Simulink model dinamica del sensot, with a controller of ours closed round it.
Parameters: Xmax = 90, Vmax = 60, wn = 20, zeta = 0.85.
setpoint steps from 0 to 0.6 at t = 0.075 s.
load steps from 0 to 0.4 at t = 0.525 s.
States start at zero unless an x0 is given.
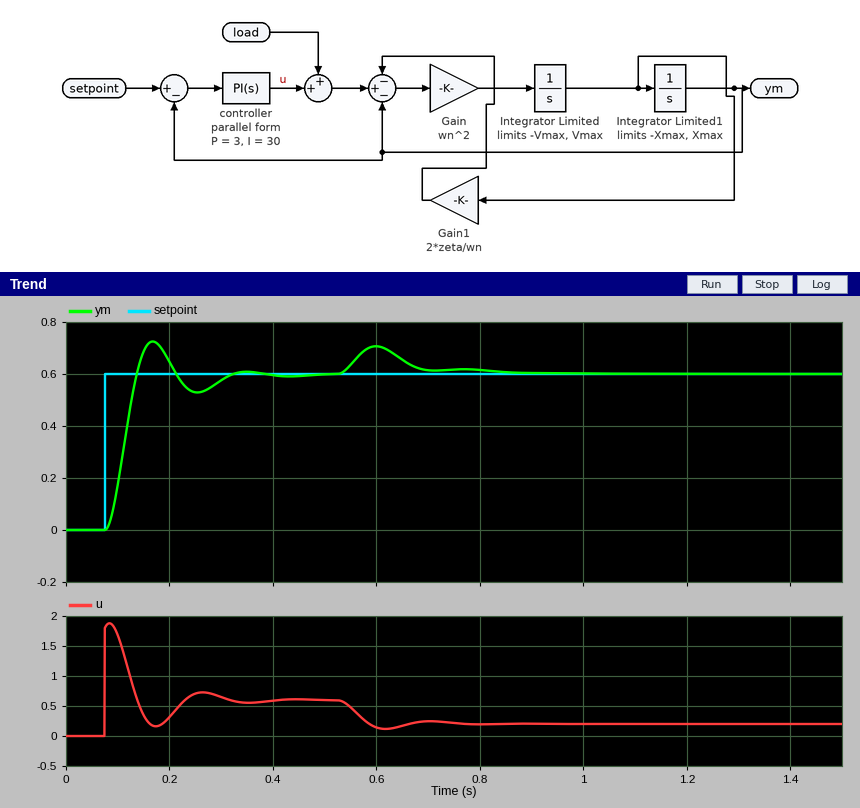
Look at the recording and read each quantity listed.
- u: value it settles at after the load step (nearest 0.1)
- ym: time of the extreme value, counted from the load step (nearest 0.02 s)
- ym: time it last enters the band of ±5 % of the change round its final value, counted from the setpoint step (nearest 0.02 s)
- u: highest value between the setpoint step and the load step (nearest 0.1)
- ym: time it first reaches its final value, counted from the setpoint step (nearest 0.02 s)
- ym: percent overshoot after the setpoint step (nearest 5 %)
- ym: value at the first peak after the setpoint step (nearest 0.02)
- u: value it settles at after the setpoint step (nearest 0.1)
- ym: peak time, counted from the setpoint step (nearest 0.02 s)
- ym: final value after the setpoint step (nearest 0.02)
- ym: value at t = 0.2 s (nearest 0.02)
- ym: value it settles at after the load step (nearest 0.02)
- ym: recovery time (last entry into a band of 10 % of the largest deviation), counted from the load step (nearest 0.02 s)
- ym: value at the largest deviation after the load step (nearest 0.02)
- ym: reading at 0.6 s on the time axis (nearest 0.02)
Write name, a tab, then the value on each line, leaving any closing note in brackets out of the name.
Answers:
u: value it settles at after the load step	0.2
ym: time of the extreme value, counted from the load step	0.08 s
ym: time it last enters the band of ±5 % of the change round its final value, counted from the setpoint step	0.22 s
u: highest value between the setpoint step and the load step	1.9
ym: time it first reaches its final value, counted from the setpoint step	0.06 s
ym: percent overshoot after the setpoint step	20 %
ym: value at the first peak after the setpoint step	0.72
u: value it settles at after the setpoint step	0.6
ym: peak time, counted from the setpoint step	0.10 s
ym: final value after the setpoint step	0.60
ym: value at t = 0.2 s	0.64
ym: value it settles at after the load step	0.60
ym: recovery time (last entry into a band of 10 % of the largest deviation), counted from the load step	0.30 s
ym: value at the largest deviation after the load step	0.70
ym: reading at 0.6 s on the time axis	0.70
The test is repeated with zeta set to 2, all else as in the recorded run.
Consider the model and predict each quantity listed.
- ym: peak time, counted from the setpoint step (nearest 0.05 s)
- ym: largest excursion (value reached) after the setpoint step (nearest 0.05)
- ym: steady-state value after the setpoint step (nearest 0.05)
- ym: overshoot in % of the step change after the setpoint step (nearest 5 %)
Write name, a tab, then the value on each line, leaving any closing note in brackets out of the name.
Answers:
ym: peak time, counted from the setpoint step	0.20 s
ym: largest excursion (value reached) after the setpoint step	0.65
ym: steady-state value after the setpoint step	0.60
ym: overshoot in % of the step change after the setpoint step	10 %
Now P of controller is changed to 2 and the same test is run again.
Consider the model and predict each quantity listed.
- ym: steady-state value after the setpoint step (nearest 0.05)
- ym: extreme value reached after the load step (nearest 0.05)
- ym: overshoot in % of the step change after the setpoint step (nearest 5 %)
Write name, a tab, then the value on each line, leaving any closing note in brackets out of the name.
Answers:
ym: steady-state value after the setpoint step	0.60
ym: extreme value reached after the load step	0.75
ym: overshoot in % of the step change after the setpoint step	25 %
